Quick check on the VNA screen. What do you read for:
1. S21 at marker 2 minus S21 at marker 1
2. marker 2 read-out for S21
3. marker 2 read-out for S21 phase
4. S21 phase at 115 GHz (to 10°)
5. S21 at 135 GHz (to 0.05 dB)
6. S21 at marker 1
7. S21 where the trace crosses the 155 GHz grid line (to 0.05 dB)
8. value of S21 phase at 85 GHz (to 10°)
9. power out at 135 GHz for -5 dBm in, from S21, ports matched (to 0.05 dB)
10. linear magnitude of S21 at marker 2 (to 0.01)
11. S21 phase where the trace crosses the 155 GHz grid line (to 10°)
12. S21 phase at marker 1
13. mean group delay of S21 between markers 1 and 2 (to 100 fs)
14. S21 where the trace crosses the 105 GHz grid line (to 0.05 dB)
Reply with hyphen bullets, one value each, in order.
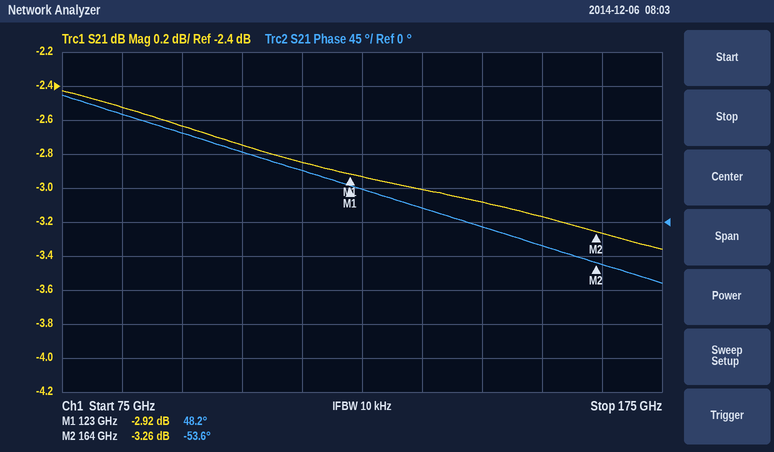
- -0.34 dB
- -3.26 dB
- -53.6°
- 70°
- -3.00 dB
- -2.92 dB
- -3.15 dB
- 140°
- -8.00 dBm
- 0.69
- -30°
- 48.2°
- 6.9 ps
- -2.75 dB
